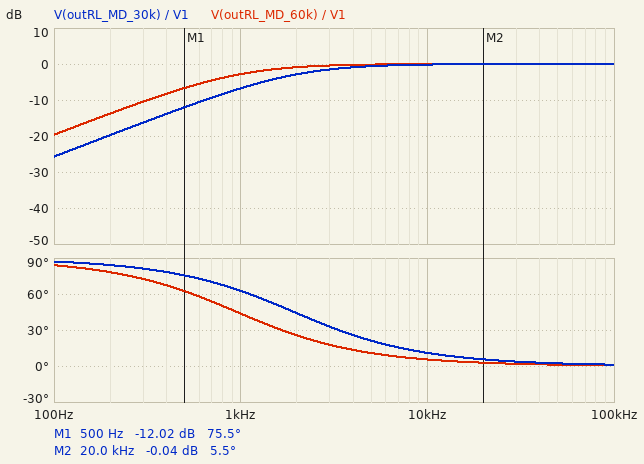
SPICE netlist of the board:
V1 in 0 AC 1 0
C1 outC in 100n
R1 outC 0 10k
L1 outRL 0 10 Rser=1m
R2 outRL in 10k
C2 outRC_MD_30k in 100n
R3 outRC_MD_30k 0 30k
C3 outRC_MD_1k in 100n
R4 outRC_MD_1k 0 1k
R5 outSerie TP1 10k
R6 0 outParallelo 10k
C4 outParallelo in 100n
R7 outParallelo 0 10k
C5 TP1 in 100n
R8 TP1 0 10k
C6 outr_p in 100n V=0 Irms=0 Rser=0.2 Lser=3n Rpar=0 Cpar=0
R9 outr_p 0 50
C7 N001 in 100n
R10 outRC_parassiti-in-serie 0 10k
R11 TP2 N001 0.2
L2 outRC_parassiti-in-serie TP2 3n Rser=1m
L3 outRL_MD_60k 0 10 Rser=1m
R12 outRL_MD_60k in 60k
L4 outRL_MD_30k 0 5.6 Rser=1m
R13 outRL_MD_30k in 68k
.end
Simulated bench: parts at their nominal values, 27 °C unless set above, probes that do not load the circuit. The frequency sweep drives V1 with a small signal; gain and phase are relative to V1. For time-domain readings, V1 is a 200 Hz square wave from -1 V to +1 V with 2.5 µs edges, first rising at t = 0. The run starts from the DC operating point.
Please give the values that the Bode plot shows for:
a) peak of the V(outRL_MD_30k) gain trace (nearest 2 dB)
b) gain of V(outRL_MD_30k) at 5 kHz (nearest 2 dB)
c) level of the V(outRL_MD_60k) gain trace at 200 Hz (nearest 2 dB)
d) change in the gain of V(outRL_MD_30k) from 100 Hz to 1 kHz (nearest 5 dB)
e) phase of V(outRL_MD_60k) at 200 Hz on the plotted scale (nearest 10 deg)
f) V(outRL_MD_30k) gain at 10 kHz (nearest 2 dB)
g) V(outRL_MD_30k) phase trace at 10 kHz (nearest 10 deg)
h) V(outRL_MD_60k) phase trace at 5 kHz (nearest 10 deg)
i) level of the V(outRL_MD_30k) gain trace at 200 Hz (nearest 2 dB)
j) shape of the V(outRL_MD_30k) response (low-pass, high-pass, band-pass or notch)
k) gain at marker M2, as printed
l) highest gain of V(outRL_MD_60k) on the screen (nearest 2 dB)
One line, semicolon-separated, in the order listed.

0 dB; 0 dB; -14 dB; 20 dB; 80 deg; 0 dB; 10 deg; 10 deg; -20 dB; high-pass; -0.04 dB; 0 dB
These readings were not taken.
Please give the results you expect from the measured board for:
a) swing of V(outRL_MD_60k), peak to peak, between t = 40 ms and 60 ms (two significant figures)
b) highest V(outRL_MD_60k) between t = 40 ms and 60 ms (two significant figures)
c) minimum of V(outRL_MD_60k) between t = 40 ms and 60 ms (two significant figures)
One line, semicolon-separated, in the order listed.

4.0 V; 2.0 V; -2.0 V
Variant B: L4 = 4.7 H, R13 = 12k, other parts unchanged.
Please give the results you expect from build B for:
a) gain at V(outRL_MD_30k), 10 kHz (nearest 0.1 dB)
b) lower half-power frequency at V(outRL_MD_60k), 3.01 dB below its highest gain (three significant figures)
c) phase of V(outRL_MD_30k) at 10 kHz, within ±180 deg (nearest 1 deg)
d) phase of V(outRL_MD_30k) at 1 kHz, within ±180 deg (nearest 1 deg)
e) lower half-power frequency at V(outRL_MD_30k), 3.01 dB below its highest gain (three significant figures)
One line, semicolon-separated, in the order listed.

0 dB; 955 Hz; 2 deg; 22 deg; 406 Hz
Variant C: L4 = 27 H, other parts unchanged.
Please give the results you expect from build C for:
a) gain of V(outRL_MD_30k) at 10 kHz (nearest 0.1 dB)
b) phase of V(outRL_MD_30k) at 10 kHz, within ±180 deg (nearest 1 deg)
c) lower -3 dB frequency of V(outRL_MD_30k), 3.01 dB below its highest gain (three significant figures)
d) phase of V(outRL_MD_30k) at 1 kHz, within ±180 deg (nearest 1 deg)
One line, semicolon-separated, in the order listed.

0 dB; 2 deg; 401 Hz; 22 deg
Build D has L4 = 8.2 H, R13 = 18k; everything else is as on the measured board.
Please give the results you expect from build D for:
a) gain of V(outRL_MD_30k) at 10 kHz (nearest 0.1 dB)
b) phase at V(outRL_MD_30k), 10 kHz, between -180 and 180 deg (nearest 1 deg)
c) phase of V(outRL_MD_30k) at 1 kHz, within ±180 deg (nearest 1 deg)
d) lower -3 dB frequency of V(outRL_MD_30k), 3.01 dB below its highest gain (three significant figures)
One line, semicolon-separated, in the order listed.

0 dB; 2 deg; 19 deg; 349 Hz
